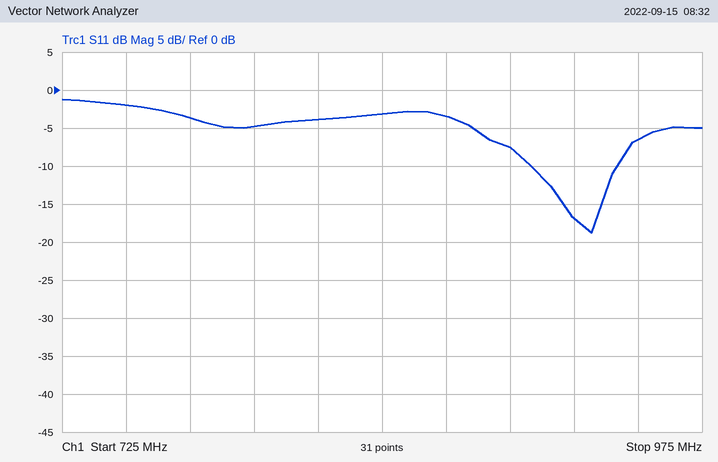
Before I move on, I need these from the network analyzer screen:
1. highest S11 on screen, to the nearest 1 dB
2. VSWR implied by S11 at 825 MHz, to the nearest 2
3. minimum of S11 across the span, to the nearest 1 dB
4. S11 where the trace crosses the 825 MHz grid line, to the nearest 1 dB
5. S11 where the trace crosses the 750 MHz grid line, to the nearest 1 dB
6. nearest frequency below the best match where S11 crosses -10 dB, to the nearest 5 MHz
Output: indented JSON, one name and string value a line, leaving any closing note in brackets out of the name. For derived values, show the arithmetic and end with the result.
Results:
{
  "highest S11 on screen, to the nearest 1 dB": "-1 dB",
  "VSWR implied by S11 at 825 MHz, to the nearest 2": "|Γ| = 10^(-4/20) = 0.6310; VSWR = (1 + 0.6310)/(1 − 0.6310) ≈ 4",
  "minimum of S11 across the span, to the nearest 1 dB": "-19 dB",
  "S11 where the trace crosses the 825 MHz grid line, to the nearest 1 dB": "-4 dB",
  "S11 where the trace crosses the 750 MHz grid line, to the nearest 1 dB": "-2 dB",
  "nearest frequency below the best match where S11 crosses -10 dB, to the nearest 5 MHz": "910 MHz"
}
